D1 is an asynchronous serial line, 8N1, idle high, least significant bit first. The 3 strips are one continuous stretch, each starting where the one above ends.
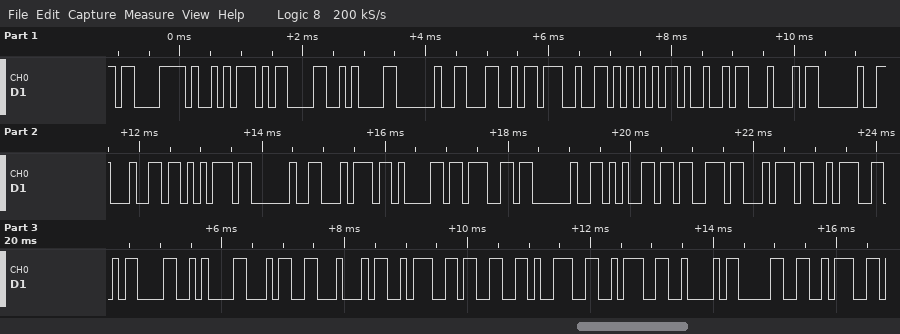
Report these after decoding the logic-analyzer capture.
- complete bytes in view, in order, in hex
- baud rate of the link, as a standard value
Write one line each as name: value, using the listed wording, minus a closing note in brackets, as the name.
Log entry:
complete bytes in view, in order, in hex: C3 A9 0D 0A 20 4C 27 55 49 44 20 64 75 20 74 61 67 20 65 73 74 3A 0D 0A 34 44 3A 33 39 3A 42 30 3A
baud rate of the link, as a standard value: 9600 baud
